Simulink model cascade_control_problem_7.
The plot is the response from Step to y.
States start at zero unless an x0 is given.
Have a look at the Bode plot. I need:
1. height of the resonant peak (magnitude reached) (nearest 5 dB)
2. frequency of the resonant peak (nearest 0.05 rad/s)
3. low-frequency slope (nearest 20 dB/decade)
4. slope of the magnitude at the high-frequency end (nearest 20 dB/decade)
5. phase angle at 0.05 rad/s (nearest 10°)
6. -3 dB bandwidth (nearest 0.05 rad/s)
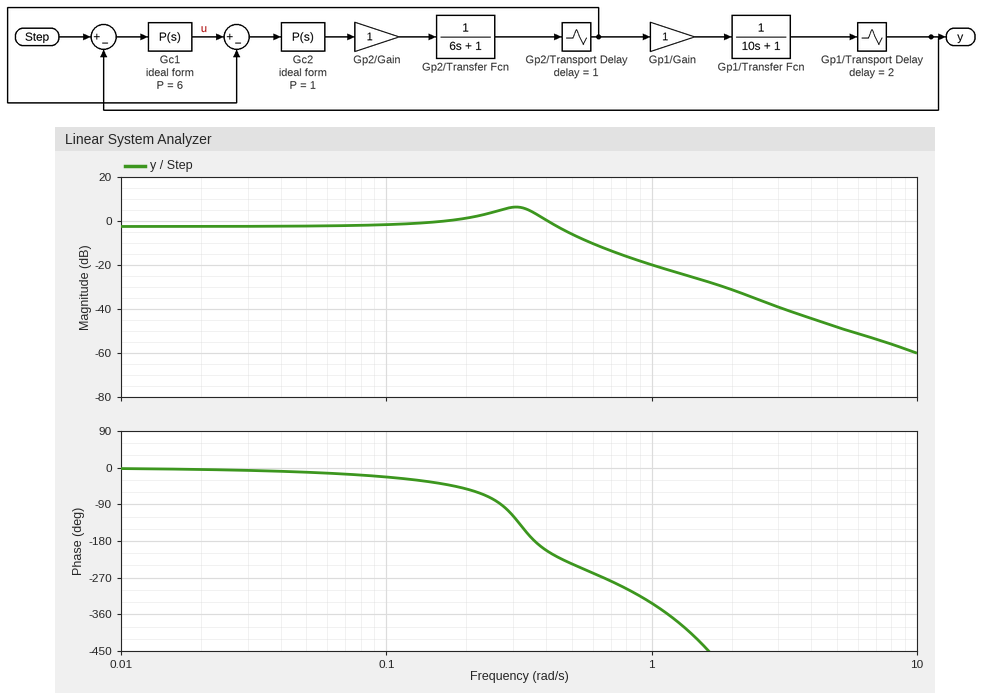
5 dB
0.30 rad/s
0 dB/decade
-40 dB/decade
-10°
0.50 rad/s
